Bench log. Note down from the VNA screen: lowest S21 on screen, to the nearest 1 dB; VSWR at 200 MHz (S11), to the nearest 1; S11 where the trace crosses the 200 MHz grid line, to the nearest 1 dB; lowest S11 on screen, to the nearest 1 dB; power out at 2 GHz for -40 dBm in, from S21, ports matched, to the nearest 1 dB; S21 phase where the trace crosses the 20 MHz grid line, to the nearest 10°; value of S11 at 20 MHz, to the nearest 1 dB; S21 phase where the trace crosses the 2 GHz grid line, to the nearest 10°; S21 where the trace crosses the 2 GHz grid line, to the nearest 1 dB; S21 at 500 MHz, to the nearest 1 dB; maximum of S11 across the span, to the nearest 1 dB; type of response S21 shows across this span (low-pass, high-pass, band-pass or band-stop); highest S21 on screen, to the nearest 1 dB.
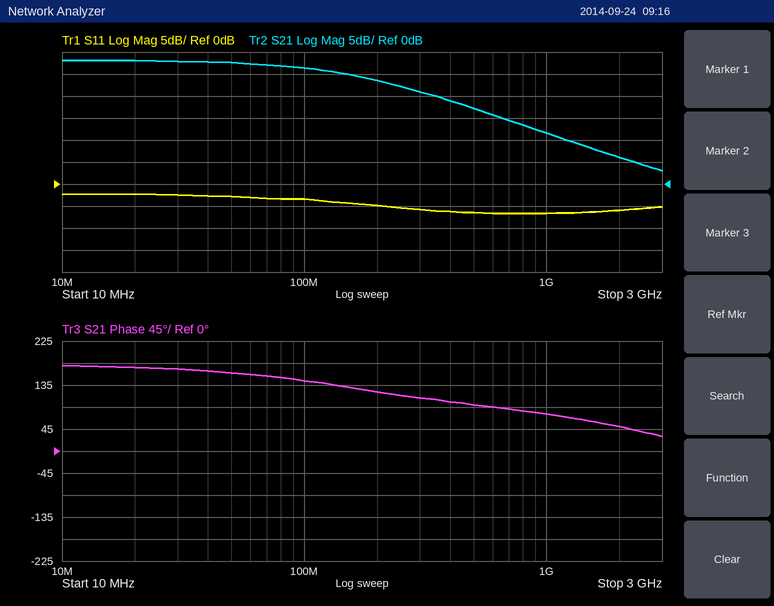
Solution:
3 dB
4
-5 dB
-7 dB
-34 dBm
170°
-2 dB
50°
6 dB
17 dB
-2 dB
low-pass
28 dB
